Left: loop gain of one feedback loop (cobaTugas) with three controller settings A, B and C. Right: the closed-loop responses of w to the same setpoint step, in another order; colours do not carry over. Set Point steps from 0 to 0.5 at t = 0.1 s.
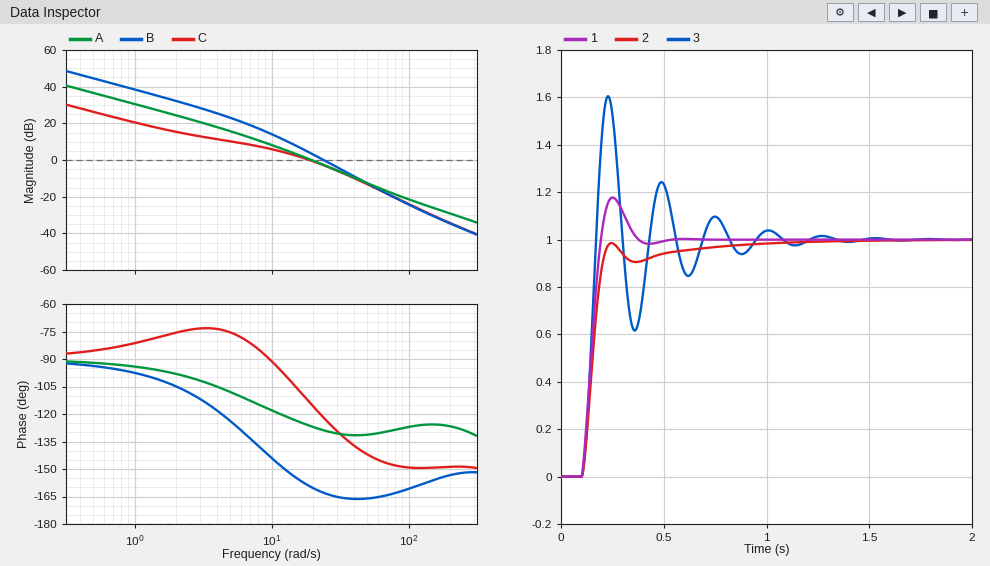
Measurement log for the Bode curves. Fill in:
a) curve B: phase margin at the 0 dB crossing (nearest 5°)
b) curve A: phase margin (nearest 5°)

15°
55°
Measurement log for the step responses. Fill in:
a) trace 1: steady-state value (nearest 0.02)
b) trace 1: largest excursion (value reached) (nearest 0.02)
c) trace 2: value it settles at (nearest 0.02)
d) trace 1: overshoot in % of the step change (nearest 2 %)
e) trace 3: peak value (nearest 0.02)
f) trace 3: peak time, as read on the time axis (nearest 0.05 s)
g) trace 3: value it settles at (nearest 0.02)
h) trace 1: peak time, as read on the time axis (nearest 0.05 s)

1.00
1.18
1.00
18 %
1.60
0.25 s
1.00
0.25 s
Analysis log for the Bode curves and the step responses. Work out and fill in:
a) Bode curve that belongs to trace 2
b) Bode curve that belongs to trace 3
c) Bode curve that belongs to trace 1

C
B
A
